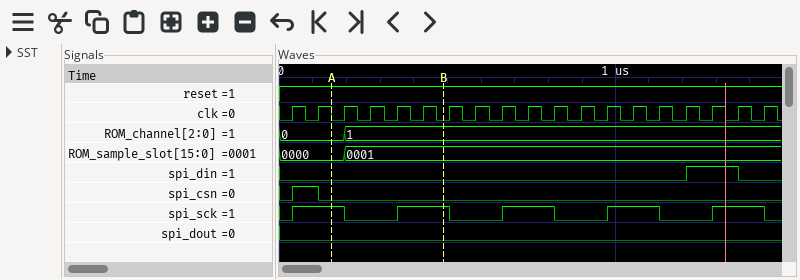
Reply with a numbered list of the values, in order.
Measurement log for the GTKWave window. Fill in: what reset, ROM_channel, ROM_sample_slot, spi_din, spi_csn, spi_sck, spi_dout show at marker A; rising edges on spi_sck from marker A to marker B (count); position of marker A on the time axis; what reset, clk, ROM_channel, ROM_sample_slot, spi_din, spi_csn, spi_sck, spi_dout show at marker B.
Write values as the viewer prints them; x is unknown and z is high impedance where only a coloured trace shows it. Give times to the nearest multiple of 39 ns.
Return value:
1. reset=1, ROM_channel=0, ROM_sample_slot=0000, spi_din=0, spi_csn=0, spi_sck=1, spi_dout=0
2. 1
3. 156 ns
4. reset=1, clk=0, ROM_channel=1, ROM_sample_slot=0001, spi_din=0, spi_csn=0, spi_sck=1, spi_dout=0
